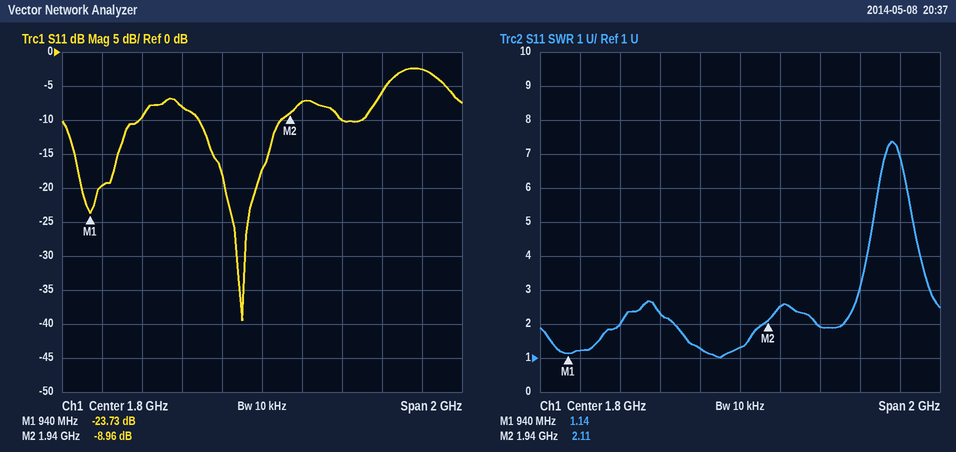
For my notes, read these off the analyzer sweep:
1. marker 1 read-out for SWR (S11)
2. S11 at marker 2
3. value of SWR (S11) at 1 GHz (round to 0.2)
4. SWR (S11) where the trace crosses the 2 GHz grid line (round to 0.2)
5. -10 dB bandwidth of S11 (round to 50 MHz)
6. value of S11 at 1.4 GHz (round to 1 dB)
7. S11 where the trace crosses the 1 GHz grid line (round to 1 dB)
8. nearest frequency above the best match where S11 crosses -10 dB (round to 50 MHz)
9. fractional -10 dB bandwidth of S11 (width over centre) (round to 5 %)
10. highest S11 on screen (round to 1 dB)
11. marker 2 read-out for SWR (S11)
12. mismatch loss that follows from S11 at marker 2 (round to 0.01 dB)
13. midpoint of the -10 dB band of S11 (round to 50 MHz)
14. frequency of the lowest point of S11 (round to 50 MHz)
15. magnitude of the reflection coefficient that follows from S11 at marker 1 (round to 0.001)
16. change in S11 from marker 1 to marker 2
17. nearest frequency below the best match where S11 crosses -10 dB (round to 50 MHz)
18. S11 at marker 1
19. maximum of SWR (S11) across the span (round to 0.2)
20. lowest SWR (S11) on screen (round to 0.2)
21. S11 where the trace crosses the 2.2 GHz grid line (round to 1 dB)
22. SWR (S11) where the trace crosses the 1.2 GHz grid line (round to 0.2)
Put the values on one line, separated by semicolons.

1.14; -8.96 dB; 1.2; 2.6; 400 MHz; -8 dB; -20 dB; 1.90 GHz; 25 %; -2 dB; 2.11; 0.59 dB; 1.70 GHz; 1.70 GHz; 0.065; 14.77 dB; 1.50 GHz; -23.73 dB; 7.4; 1.0; -10 dB; 2.0
